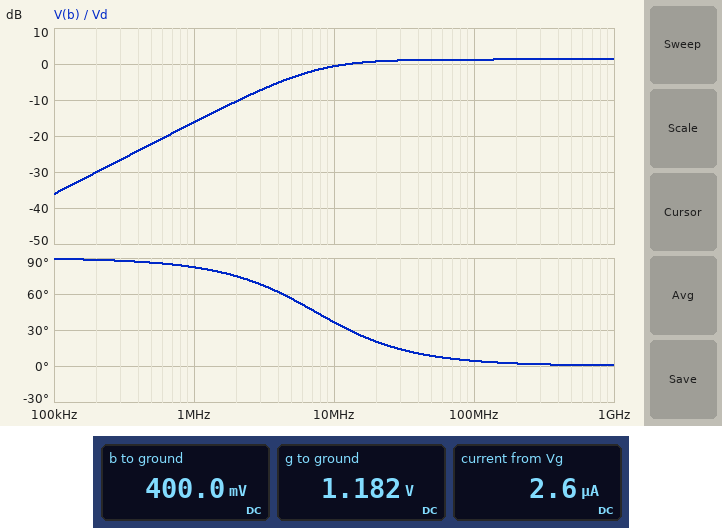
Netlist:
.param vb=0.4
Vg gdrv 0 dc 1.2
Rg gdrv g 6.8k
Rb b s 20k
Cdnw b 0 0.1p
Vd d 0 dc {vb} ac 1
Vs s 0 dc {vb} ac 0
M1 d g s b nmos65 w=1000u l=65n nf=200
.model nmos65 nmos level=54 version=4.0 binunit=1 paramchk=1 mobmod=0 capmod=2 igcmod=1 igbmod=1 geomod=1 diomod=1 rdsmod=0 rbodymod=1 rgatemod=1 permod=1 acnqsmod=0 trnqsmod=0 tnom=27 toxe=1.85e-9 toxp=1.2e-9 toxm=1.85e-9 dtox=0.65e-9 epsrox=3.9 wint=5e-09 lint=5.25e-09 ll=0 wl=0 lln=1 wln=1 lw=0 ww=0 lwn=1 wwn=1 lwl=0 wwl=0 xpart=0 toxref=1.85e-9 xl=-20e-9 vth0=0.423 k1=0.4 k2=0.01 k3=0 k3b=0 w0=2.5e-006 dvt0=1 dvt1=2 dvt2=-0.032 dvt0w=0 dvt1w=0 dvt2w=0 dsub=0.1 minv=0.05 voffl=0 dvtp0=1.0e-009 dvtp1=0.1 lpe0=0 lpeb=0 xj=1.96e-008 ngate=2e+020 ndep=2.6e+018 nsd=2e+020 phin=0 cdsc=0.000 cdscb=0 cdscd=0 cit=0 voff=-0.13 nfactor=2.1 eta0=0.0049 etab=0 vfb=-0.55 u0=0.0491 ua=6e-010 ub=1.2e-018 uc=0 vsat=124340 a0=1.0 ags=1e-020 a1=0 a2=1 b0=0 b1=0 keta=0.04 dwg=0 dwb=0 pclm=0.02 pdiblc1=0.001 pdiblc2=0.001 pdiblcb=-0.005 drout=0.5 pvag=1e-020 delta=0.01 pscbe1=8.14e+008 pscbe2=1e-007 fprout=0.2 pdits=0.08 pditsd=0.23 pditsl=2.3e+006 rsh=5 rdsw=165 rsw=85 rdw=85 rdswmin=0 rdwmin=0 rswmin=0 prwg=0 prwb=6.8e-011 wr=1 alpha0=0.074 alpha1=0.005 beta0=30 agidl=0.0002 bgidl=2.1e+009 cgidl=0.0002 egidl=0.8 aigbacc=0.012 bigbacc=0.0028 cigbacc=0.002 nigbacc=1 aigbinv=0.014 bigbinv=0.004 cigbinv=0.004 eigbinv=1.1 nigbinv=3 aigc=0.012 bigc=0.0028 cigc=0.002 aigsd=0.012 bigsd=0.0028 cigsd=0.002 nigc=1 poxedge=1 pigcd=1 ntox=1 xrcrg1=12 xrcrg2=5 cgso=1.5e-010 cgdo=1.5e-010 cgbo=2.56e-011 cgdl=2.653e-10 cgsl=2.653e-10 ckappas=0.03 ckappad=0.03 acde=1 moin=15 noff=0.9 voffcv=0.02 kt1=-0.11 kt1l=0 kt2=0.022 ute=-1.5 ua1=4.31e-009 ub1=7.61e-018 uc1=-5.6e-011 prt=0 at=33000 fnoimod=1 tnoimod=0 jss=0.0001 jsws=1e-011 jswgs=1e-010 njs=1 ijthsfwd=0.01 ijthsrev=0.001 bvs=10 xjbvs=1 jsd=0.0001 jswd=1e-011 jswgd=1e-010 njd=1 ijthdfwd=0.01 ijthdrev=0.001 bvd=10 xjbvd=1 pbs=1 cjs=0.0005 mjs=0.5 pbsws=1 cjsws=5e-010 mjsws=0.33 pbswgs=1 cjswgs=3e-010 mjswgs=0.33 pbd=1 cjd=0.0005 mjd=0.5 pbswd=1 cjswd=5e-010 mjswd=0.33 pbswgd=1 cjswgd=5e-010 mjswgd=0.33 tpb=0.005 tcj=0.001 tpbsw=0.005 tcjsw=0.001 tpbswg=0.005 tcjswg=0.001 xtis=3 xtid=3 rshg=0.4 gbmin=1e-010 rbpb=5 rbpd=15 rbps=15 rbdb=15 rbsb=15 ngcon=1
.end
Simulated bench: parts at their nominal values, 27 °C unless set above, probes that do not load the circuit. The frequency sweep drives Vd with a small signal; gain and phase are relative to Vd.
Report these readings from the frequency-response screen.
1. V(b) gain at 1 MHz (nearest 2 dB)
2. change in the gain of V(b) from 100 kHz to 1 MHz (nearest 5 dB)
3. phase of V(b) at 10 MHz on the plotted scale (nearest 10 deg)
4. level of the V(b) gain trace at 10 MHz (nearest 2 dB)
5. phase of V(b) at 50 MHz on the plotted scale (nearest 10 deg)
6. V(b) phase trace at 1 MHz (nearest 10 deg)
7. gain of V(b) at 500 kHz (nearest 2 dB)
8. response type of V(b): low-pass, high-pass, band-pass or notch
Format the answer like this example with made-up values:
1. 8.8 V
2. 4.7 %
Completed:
1. -16 dB
2. 20 dB
3. 40 deg
4. 0 dB
5. 10 deg
6. 80 deg
7. -22 dB
8. high-pass
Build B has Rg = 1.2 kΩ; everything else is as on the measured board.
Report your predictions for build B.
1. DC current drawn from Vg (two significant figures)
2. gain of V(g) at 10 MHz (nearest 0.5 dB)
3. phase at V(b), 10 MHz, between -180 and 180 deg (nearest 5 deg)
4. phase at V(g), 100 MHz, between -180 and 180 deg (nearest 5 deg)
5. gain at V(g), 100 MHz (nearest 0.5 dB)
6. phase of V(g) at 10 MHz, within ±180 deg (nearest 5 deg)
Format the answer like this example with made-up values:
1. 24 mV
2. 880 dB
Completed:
1. 2.9 µA
2. -24.0 dB
3. 35 deg
4. 35 deg
5. -8.5 dB
6. 80 deg
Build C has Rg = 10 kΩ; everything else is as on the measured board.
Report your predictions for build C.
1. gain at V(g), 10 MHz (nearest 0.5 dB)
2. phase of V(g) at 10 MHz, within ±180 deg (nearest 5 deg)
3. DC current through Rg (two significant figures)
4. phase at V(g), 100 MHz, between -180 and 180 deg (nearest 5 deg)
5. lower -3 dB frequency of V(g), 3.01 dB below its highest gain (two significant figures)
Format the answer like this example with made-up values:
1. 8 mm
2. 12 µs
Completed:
1. -10.0 dB
2. 40 deg
3. 2.5 µA
4. 5 deg
5. 10 MHz
